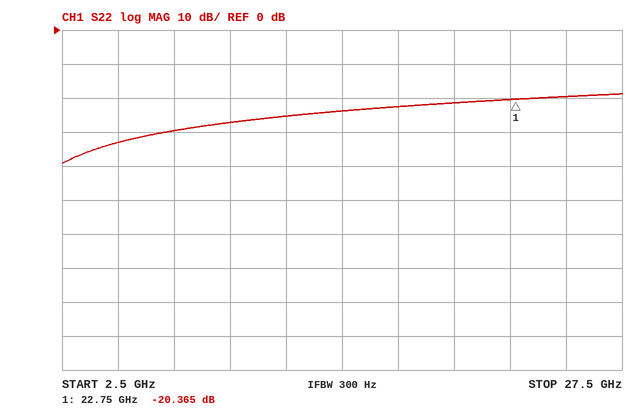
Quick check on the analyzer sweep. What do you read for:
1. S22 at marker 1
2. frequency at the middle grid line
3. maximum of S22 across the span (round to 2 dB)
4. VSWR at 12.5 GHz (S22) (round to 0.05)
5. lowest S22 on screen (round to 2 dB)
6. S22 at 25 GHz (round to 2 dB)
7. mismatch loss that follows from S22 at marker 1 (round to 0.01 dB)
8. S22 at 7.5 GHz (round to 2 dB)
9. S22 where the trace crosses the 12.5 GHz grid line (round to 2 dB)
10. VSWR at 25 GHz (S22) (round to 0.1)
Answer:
-20.365 dB
15 GHz
-18 dB
1.10
-40 dB
-20 dB
0.04 dB
-30 dB
-26 dB
1.2
